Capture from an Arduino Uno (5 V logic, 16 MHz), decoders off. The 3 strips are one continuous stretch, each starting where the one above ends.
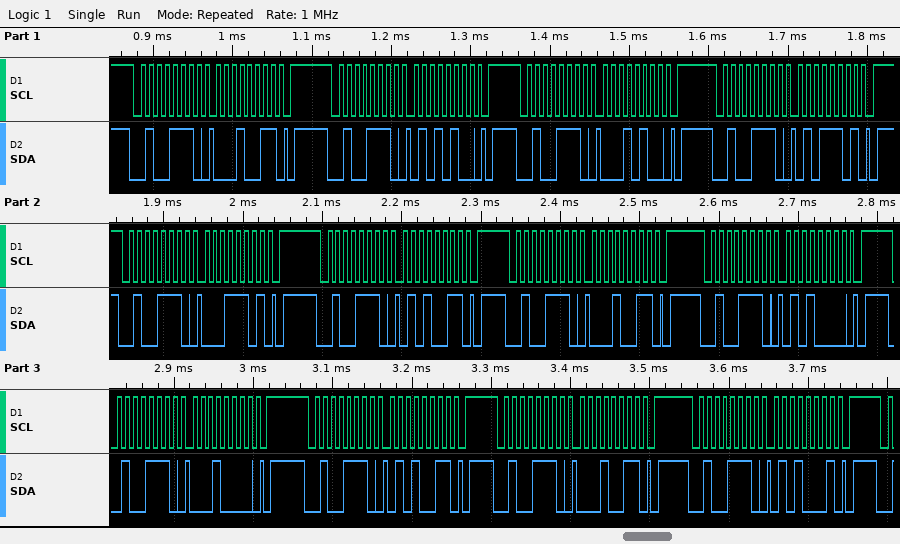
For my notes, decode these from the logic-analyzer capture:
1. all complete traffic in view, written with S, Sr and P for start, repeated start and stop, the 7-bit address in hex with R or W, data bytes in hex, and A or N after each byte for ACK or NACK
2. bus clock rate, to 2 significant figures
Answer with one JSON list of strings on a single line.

["S 27W A 13 A P S 27W A 54 A P S 27W A 14 A P S 27W A 5D A P S 27W A 1D A P S 27W A 53 A P S 27W A 13 A P S 27W A 50 A P S 27W A 10 A P S 27W A 53 A P S 27W A 13 A P S 27W A 51 A P", "100 kHz"]
